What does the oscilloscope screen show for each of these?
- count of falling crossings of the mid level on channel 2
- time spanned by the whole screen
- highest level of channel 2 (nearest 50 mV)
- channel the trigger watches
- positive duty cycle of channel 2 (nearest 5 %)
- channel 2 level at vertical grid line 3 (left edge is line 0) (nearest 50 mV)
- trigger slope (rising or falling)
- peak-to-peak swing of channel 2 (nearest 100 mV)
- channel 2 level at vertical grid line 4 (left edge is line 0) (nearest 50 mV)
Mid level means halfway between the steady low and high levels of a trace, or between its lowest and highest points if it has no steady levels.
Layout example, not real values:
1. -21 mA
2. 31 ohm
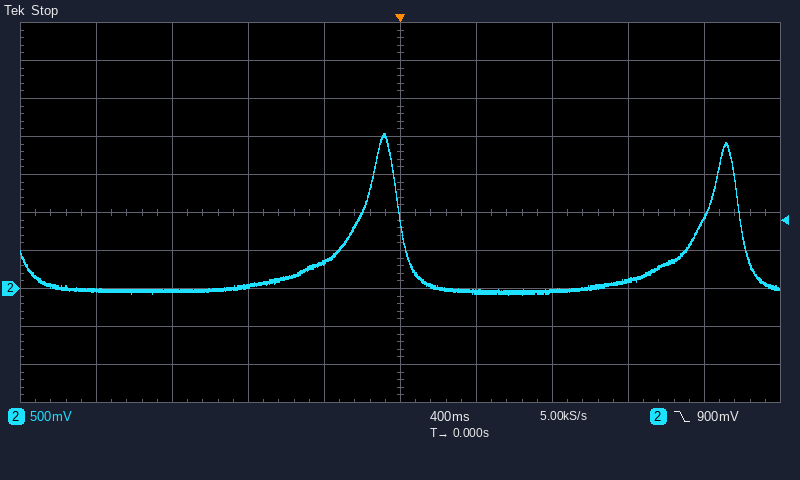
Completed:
1. 2
2. 4 s
3. 2.05 V
4. channel 2
5. 10 %
6. 50 mV
7. falling
8. 2.10 V
9. 350 mV
